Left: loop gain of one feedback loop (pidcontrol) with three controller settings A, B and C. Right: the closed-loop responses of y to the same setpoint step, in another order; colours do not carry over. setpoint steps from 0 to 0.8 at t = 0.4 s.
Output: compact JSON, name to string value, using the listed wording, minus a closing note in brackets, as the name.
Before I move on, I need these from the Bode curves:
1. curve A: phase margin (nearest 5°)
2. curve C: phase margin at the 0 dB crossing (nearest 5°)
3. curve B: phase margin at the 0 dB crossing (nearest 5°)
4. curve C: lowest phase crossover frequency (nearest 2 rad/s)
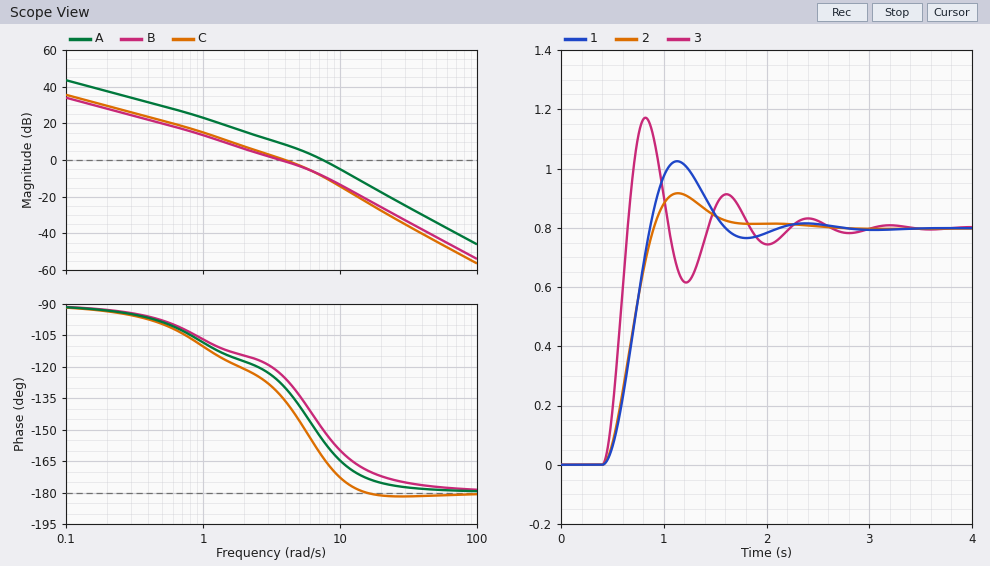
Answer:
{"curve A: phase margin": "25°", "curve C: phase margin at the 0 dB crossing": "45°", "curve B: phase margin at the 0 dB crossing": "55°", "curve C: lowest phase crossover frequency": "16 rad/s"}
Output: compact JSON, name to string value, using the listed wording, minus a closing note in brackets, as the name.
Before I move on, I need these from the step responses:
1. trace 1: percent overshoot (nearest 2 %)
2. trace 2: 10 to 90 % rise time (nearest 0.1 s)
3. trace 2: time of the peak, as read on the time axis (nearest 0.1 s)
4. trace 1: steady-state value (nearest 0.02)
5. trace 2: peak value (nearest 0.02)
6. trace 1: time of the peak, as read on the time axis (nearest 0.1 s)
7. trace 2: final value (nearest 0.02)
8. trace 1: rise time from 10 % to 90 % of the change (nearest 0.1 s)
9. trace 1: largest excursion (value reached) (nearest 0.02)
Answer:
{"trace 1: percent overshoot": "28 %", "trace 2: 10 to 90 % rise time": "0.3 s", "trace 2: time of the peak, as read on the time axis": "1.1 s", "trace 1: steady-state value": "0.80", "trace 2: peak value": "0.92", "trace 1: time of the peak, as read on the time axis": "1.1 s", "trace 2: final value": "0.80", "trace 1: rise time from 10 % to 90 % of the change": "0.3 s", "trace 1: largest excursion (value reached)": "1.02"}
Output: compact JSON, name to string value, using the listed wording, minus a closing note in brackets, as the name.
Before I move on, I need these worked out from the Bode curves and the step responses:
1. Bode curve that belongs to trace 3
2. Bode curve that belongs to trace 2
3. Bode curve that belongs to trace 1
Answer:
{"Bode curve that belongs to trace 3": "A", "Bode curve that belongs to trace 2": "B", "Bode curve that belongs to trace 1": "C"}
